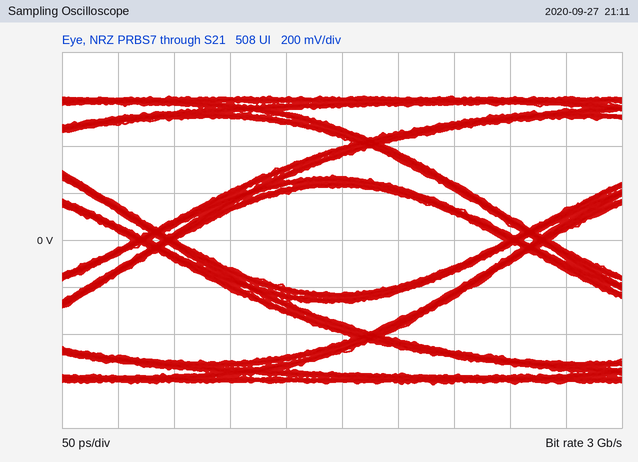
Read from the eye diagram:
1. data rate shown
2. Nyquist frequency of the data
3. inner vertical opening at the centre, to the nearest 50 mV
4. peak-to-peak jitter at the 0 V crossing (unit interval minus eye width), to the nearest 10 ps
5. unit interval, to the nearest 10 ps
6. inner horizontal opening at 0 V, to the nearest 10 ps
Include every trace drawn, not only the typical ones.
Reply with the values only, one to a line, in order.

3 Gb/s
1.5 GHz
450 mV
40 ps
330 ps
290 ps
